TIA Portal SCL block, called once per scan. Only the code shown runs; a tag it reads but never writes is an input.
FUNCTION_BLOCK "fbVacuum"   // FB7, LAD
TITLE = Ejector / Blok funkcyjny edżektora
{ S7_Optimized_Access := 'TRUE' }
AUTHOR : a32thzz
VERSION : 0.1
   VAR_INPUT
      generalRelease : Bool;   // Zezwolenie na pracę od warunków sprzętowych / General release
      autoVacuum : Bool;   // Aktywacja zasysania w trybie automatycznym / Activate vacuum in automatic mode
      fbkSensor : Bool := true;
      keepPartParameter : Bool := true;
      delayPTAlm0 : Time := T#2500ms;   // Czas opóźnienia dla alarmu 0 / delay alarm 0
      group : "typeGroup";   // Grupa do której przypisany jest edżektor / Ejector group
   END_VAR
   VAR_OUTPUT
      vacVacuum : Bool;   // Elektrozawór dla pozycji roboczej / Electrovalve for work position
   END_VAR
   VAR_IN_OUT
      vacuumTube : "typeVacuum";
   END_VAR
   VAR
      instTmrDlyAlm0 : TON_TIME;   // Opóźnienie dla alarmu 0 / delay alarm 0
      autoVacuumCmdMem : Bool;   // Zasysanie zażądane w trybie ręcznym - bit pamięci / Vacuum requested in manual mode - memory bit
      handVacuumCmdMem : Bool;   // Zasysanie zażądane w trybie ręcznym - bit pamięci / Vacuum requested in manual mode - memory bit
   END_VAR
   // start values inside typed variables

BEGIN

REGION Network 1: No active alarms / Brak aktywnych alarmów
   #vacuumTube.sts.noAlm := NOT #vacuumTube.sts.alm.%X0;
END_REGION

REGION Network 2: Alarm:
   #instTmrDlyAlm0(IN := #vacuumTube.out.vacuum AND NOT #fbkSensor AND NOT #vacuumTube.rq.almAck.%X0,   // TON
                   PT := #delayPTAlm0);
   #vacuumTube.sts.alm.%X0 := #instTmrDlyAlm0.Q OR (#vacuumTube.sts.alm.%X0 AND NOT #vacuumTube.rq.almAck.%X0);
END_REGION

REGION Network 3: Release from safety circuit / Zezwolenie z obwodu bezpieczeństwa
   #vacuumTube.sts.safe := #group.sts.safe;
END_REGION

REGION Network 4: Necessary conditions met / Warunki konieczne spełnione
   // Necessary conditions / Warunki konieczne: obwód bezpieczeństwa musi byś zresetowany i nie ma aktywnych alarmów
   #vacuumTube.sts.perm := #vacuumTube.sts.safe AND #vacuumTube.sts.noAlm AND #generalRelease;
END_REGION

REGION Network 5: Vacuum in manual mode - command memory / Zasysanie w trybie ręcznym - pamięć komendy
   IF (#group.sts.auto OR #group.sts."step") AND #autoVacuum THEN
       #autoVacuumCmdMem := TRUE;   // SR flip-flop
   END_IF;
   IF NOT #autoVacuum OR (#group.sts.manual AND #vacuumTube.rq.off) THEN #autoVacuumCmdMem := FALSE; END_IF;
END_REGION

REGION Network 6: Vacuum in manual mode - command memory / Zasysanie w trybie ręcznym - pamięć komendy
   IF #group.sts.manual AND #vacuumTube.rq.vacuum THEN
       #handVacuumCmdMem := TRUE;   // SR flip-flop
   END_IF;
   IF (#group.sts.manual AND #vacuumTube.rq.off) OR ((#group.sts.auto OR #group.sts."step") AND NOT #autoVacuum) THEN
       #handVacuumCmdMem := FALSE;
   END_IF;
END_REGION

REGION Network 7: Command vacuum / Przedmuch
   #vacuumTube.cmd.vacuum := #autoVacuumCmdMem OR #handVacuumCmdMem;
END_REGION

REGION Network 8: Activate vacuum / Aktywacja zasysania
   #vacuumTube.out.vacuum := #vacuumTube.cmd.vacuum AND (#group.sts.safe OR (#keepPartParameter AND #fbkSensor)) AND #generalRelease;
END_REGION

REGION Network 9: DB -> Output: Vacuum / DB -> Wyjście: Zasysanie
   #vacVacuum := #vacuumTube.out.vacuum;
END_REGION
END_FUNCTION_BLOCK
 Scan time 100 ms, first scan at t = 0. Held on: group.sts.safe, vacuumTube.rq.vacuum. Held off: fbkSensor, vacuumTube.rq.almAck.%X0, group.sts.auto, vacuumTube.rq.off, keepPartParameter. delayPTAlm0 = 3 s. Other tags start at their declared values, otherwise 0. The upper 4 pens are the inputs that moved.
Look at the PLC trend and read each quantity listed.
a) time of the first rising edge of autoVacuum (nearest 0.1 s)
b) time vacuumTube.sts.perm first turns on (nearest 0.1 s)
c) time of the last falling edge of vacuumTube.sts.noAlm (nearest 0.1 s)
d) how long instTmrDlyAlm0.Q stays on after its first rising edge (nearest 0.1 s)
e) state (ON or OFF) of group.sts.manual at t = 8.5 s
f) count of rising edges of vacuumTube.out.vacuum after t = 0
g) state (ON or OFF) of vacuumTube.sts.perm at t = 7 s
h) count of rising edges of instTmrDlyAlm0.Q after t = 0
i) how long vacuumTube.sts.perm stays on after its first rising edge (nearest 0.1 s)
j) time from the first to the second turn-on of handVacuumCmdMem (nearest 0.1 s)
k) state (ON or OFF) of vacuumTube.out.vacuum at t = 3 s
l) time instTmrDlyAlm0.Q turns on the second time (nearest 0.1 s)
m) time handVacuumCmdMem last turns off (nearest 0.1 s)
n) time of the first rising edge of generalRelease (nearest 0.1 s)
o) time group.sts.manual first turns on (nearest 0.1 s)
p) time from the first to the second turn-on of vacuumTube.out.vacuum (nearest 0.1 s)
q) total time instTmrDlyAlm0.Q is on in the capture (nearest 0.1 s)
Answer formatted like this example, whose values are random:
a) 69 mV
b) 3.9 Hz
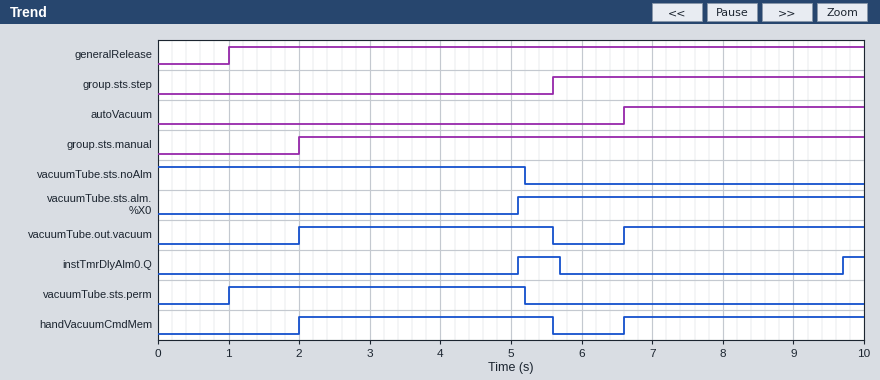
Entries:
a) 6.6 s
b) 1.0 s
c) 5.2 s
d) 0.6 s
e) ON
f) 2
g) OFF
h) 2
i) 4.2 s
j) 4.6 s
k) ON
l) 9.7 s
m) 5.6 s
n) 1.0 s
o) 2.0 s
p) 4.6 s
q) 0.9 s
